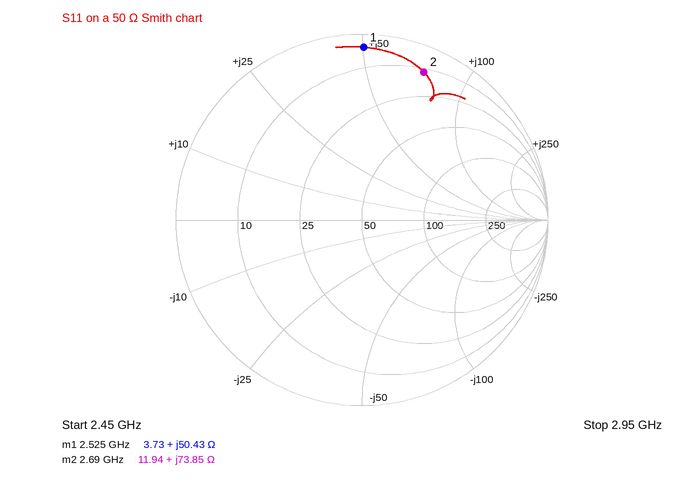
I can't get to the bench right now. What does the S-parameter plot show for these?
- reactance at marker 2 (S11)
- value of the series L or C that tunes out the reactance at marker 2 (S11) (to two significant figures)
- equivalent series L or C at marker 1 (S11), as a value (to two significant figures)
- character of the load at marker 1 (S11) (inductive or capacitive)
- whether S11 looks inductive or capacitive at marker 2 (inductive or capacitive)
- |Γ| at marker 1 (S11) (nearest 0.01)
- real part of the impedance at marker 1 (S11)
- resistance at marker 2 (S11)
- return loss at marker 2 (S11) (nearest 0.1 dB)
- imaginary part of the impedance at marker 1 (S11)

+73.85 Ω
800 fF
3.2 nH
inductive
inductive
0.93
3.73 Ω
11.94 Ω
1.3 dB
+50.43 Ω
